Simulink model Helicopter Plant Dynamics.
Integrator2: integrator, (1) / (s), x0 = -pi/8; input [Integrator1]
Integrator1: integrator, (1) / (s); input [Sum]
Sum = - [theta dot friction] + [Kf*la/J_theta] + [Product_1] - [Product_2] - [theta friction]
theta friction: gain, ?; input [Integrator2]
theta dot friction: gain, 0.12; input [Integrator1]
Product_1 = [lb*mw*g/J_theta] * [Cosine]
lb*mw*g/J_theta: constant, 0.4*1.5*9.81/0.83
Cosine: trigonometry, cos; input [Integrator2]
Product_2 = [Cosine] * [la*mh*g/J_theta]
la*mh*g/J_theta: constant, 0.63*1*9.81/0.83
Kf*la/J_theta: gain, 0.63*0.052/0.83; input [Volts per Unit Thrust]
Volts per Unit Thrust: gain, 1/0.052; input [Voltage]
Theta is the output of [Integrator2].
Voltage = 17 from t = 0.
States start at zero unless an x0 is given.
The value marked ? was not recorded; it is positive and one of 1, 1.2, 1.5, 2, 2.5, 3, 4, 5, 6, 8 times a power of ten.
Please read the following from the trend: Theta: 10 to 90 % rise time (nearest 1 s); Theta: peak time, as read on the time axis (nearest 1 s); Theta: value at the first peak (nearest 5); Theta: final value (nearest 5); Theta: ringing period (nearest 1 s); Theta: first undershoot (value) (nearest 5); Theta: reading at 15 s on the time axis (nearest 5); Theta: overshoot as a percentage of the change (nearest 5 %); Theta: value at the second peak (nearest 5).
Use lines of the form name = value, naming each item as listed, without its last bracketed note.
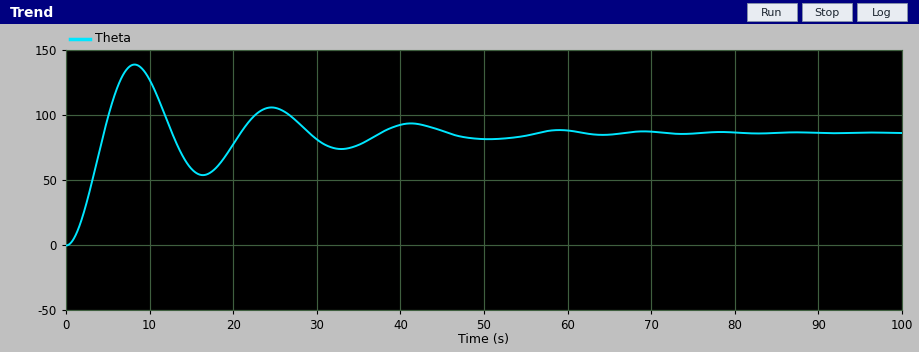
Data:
Theta: 10 to 90 % rise time = 3 s
Theta: peak time, as read on the time axis = 8 s
Theta: value at the first peak = 140
Theta: final value = 85
Theta: ringing period = 16 s
Theta: first undershoot (value) = 55
Theta: reading at 15 s on the time axis = 60
Theta: overshoot as a percentage of the change = 60 %
Theta: value at the second peak = 105
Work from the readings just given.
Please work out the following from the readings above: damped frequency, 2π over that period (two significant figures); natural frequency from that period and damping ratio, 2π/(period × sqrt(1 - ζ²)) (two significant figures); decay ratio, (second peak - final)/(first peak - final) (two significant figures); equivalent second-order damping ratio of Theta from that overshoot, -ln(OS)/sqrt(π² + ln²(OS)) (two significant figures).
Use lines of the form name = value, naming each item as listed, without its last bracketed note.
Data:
damped frequency, 2π over that period = 0.39 rad/s
natural frequency from that period and damping ratio, 2π/(period × sqrt(1 - ζ²)) = 0.40 rad/s
decay ratio, (second peak - final)/(first peak - final) = 0.36
equivalent second-order damping ratio of Theta from that overshoot, -ln(OS)/sqrt(π² + ln²(OS)) = 0.16
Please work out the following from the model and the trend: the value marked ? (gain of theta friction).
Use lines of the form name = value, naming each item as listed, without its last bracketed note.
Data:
the value marked ? = 0.15
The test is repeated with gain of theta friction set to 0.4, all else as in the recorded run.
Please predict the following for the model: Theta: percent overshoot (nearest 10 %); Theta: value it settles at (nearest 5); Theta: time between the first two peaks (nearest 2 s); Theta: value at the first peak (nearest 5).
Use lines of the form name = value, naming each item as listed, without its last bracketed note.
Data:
Theta: percent overshoot = 80 %
Theta: value it settles at = 30
Theta: time between the first two peaks = 10 s
Theta: value at the first peak = 55
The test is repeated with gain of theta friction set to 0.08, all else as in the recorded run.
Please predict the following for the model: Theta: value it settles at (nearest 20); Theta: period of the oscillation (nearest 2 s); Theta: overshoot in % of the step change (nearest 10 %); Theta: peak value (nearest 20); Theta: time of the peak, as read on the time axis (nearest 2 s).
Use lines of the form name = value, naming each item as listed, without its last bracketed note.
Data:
Theta: value it settles at = 160
Theta: period of the oscillation = 22 s
Theta: overshoot in % of the step change = 50 %
Theta: peak value = 240
Theta: time of the peak, as read on the time axis = 12 s
